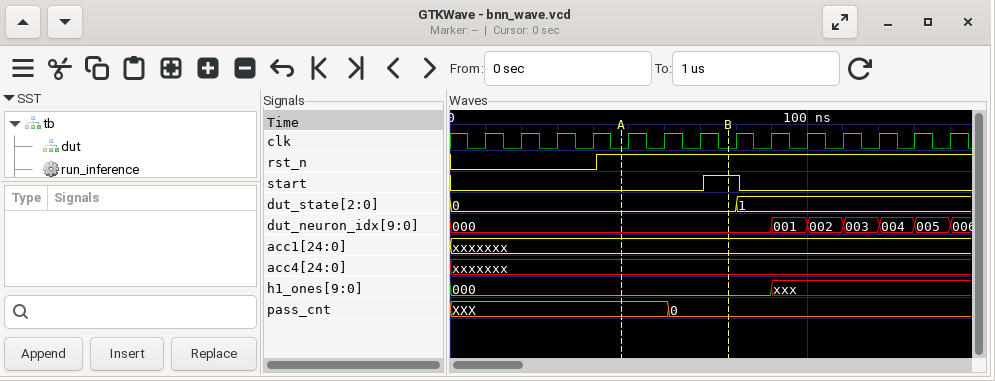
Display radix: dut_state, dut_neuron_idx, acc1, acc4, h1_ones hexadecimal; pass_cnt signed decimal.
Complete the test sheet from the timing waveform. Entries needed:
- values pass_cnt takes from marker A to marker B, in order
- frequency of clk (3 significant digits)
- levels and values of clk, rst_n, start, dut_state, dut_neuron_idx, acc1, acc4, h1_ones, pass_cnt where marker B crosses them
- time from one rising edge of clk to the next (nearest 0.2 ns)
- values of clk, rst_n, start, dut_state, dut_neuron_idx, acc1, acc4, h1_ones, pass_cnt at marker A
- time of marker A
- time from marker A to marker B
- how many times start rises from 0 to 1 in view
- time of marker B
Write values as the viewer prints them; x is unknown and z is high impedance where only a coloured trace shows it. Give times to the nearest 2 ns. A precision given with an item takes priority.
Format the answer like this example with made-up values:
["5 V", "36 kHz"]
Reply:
["XXX, 0", "100 MHz", "clk=0, rst_n=1, start=1, dut_state=0, dut_neuron_idx=000, acc1=xxxxxxx, acc4=xxxxxxx, h1_ones=000, pass_cnt=0", "10 ns", "clk=0, rst_n=1, start=0, dut_state=0, dut_neuron_idx=000, acc1=xxxxxxx, acc4=xxxxxxx, h1_ones=000, pass_cnt=XXX", "48 ns", "30 ns", "1", "78 ns"]
